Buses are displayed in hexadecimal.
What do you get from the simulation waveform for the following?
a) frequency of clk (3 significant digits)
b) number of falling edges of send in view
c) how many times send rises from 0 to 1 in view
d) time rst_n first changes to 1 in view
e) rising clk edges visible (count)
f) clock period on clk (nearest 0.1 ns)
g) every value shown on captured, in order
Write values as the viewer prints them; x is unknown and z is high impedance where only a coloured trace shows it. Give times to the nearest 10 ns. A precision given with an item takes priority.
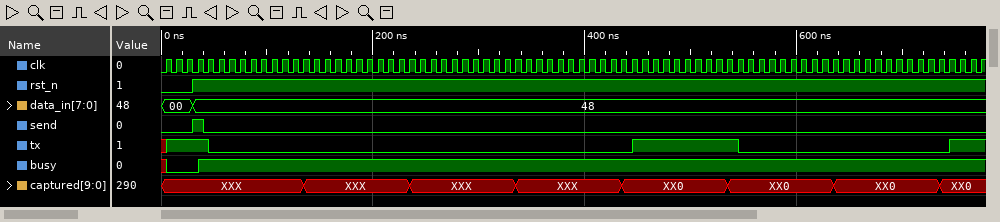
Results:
100 MHz
1
1
30 ns
78
10 ns
XXX, XXX, XXX, XXX, XX0, XX0, XX0, XX0
